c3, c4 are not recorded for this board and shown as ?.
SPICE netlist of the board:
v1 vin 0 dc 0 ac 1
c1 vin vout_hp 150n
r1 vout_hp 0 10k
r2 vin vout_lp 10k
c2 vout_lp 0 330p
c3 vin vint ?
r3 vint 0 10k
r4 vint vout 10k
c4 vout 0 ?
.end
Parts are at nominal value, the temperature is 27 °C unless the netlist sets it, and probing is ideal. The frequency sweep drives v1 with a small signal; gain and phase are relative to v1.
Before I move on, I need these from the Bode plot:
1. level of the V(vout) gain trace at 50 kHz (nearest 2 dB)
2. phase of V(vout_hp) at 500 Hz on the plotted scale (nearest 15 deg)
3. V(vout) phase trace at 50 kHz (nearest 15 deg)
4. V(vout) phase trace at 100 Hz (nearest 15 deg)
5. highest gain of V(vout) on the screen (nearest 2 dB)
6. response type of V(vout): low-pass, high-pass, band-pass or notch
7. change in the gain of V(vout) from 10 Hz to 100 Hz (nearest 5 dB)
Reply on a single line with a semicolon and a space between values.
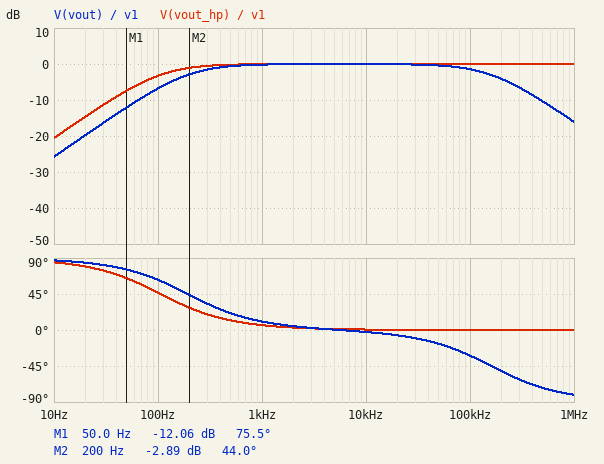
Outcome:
0 dB; 15 deg; -15 deg; 60 deg; 0 dB; band-pass; 20 dB
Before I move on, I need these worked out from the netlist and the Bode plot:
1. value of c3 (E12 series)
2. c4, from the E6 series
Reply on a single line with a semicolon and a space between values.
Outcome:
82 nF; 100 pF
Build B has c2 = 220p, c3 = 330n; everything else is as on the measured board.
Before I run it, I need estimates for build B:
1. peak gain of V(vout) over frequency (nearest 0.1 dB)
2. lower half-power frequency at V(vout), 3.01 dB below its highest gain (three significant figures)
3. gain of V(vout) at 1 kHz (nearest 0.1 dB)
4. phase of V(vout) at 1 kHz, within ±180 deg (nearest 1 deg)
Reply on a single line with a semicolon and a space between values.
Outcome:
0 dB; 48.2 Hz; 0 dB; 2 deg
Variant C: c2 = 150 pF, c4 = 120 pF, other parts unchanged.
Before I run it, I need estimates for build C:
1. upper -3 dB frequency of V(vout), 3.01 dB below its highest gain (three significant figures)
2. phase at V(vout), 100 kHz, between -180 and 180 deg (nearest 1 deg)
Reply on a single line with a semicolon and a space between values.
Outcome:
133 kHz; -37 deg
